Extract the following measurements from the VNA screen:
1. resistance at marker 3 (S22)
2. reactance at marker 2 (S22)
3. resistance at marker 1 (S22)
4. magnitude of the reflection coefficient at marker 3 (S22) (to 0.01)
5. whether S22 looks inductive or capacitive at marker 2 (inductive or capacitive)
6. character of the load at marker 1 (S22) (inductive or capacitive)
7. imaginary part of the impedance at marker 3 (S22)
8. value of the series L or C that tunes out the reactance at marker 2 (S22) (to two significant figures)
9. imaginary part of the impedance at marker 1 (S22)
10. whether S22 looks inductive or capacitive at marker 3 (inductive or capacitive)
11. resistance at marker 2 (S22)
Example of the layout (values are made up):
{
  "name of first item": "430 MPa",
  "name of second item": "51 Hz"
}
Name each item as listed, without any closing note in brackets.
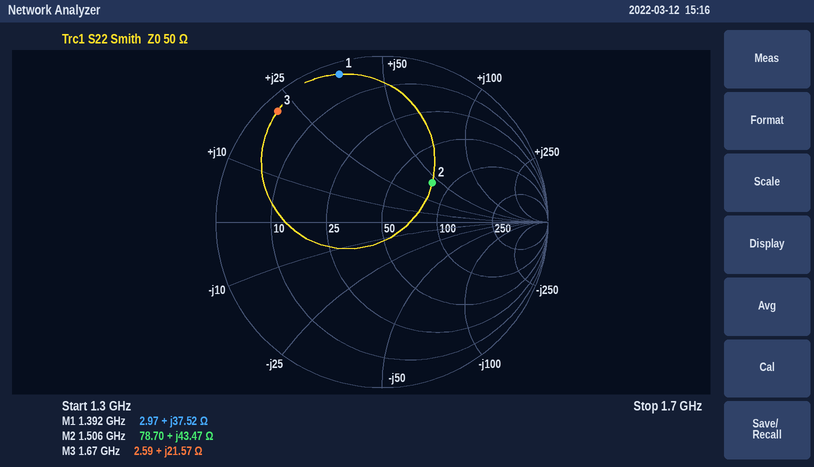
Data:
{
  "resistance at marker 3": "2.59 Ω",
  "reactance at marker 2": "+43.47 Ω",
  "resistance at marker 1": "2.97 Ω",
  "magnitude of the reflection coefficient at marker 3 (S22)": "0.92",
  "whether S22 looks inductive or capacitive at marker 2": "inductive",
  "character of the load at marker 1 (S22)": "inductive",
  "imaginary part of the impedance at marker 3": "+21.57 Ω",
  "value of the series L or C that tunes out the reactance at marker 2 (S22)": "2.4 pF",
  "imaginary part of the impedance at marker 1": "+37.52 Ω",
  "whether S22 looks inductive or capacitive at marker 3": "inductive",
  "resistance at marker 2": "78.70 Ω"
}
